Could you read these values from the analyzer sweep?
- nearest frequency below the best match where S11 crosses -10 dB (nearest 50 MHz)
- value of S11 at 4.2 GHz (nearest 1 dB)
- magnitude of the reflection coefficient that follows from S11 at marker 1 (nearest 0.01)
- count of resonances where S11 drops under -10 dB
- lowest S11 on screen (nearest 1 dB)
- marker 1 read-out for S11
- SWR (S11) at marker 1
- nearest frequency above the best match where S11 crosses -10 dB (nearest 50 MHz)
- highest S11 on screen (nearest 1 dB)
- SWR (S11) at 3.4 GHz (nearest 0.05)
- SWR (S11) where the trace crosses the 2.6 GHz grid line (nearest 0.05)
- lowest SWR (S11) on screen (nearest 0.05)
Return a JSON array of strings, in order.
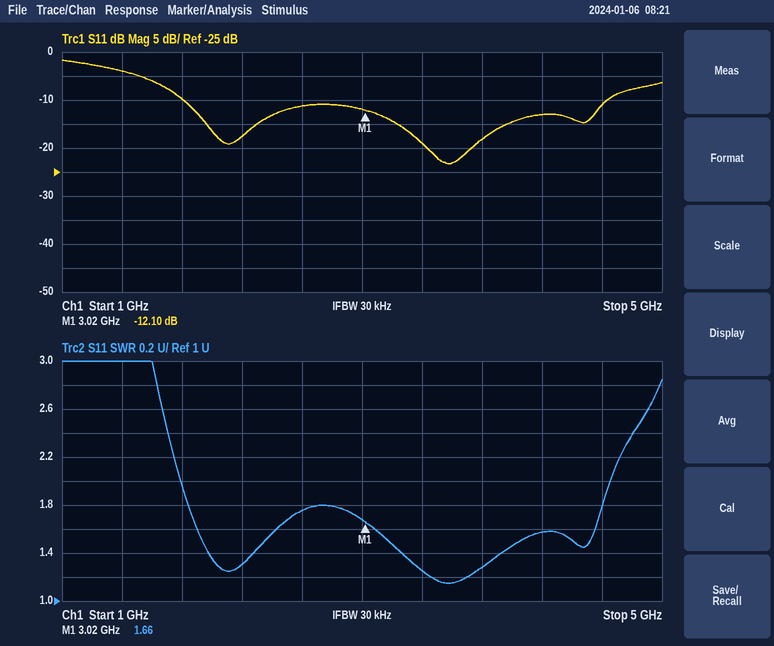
["1.80 GHz", "-13 dB", "0.25", "2", "-23 dB", "-12.10 dB", "1.66", "4.65 GHz", "-2 dB", "1.25", "1.75", "1.15"]
